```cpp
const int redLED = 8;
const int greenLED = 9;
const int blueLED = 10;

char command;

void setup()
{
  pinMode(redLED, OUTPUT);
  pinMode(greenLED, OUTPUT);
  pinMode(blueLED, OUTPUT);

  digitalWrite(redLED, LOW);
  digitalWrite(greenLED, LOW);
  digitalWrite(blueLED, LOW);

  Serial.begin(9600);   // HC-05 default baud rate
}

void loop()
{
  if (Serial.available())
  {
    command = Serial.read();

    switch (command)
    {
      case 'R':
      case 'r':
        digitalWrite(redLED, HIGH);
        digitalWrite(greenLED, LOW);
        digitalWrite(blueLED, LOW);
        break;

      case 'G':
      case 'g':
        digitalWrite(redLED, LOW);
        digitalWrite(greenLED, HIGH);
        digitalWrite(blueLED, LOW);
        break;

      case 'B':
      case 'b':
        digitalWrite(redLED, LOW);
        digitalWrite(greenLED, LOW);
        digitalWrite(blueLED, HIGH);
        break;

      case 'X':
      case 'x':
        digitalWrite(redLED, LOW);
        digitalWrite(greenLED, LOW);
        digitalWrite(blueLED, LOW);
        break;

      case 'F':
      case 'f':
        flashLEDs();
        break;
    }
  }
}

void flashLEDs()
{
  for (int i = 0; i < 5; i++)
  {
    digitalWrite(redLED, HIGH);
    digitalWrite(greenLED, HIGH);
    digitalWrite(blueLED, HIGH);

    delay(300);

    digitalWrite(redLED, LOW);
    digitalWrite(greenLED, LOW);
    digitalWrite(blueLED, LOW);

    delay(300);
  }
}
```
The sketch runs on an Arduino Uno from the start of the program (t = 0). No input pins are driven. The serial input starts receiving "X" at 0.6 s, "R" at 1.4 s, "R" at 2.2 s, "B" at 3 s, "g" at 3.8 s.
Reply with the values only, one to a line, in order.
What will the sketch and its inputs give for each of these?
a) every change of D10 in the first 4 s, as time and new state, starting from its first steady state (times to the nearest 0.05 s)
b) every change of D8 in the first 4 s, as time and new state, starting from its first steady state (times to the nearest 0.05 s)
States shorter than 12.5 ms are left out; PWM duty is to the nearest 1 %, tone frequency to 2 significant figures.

0 s low; 3 s high; 3.8 s low
0 s low; 1.4 s high; 3 s low
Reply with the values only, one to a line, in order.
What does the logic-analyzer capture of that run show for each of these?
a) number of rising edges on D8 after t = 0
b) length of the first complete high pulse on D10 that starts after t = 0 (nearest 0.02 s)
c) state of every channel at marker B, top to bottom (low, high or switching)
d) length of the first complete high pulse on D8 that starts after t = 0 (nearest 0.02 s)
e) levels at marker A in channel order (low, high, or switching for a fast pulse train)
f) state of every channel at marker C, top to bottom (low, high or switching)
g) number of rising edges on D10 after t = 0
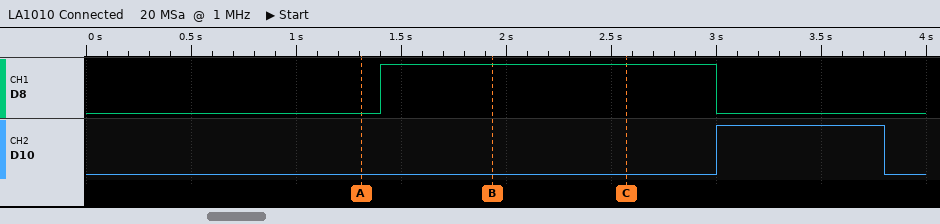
1
0.80 s
D8 high, D10 low
1.60 s
D8 low, D10 low
D8 high, D10 low
1
